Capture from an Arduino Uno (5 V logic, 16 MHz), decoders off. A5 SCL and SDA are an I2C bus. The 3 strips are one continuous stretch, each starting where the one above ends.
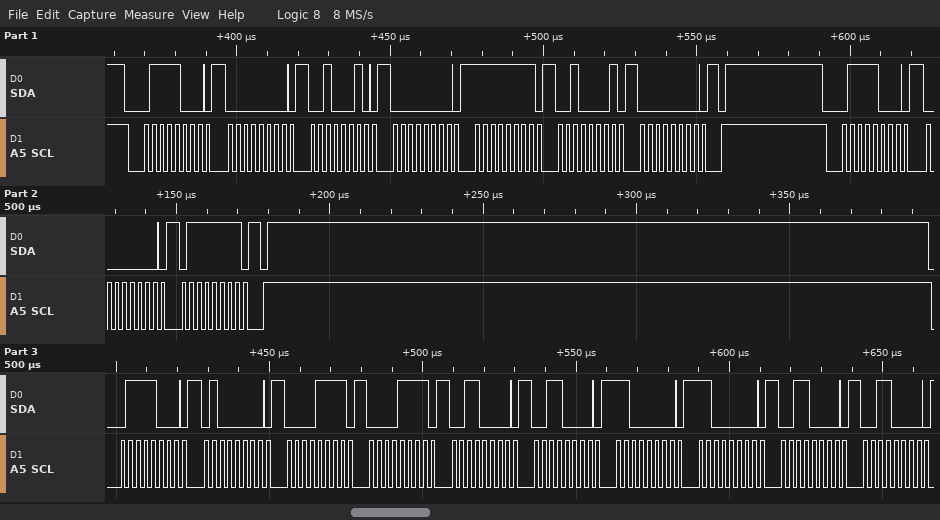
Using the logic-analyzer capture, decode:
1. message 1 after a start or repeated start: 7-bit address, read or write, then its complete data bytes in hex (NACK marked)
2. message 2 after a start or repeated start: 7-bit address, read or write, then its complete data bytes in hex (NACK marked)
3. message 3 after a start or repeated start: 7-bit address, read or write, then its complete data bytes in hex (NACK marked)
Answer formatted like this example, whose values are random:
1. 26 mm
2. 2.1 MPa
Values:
1. 0x3C write: 00 22 00 FF 21 00
2. 0x3C write: 00 7F
3. 0x3C write: 40 0F 0F 30 30 C0 C0 30 30
